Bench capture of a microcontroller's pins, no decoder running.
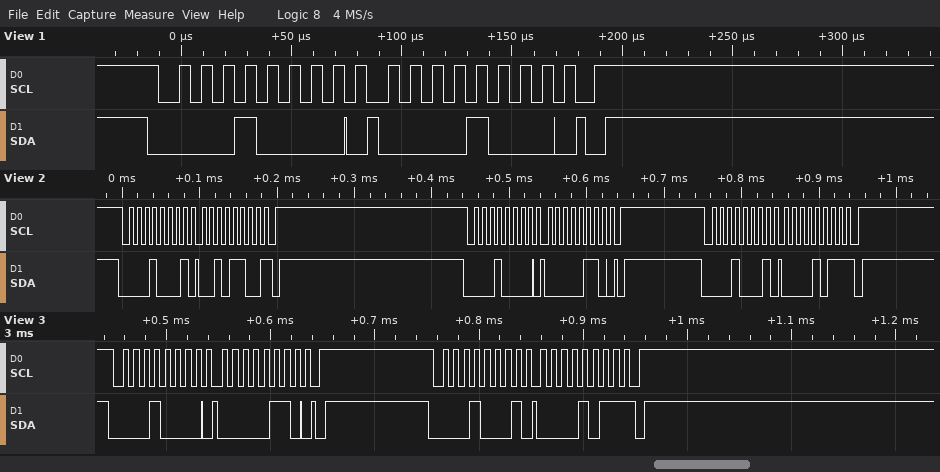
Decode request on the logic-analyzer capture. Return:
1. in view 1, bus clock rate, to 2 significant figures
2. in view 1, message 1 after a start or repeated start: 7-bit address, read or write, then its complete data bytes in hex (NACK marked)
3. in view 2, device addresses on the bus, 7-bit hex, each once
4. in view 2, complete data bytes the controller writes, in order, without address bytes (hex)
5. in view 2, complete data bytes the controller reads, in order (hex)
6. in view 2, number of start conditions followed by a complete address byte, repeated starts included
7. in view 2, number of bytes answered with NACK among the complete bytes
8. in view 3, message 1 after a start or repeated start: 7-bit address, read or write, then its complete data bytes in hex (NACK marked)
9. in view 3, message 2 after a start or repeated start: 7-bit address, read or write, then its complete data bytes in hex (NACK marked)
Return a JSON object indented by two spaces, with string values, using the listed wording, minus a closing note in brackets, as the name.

{
  "in view 1, bus clock rate, to 2 significant figures": "100 kHz",
  "in view 1, message 1 after a start or repeated start: 7-bit address, read or write, then its complete data bytes in hex": "0x08 write: 08",
  "in view 2, device addresses on the bus, 7-bit hex, each once": "0x08",
  "in view 2, complete data bytes the controller writes, in order, without address bytes": "06",
  "in view 2, complete data bytes the controller reads, in order": "2C 0B",
  "in view 2, number of start conditions followed by a complete address byte, repeated starts included": "3",
  "in view 2, number of bytes answered with NACK among the complete bytes": "2",
  "in view 3, message 1 after a start or repeated start: 7-bit address, read or write, then its complete data bytes in hex": "0x08 write: 06",
  "in view 3, message 2 after a start or repeated start: 7-bit address, read or write, then its complete data bytes in hex": "0x08 read: 0B NACK"
}
